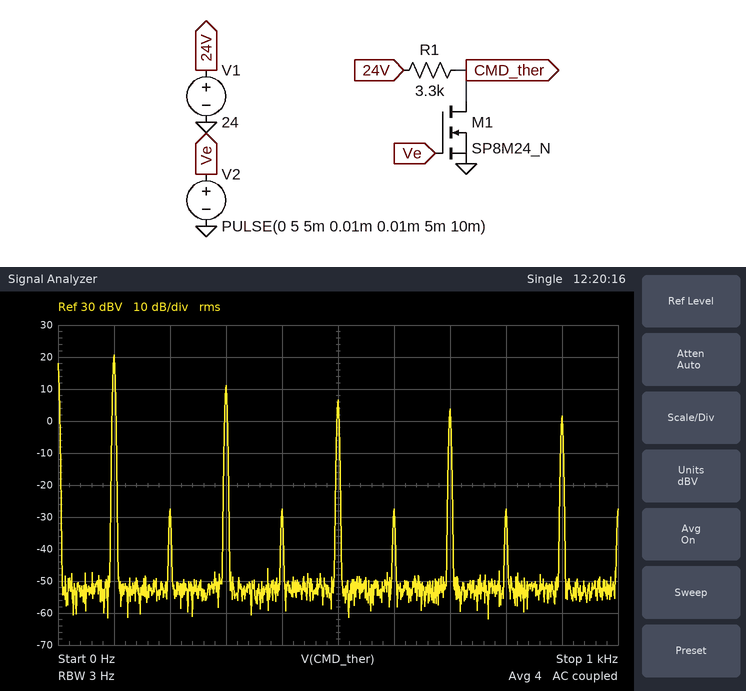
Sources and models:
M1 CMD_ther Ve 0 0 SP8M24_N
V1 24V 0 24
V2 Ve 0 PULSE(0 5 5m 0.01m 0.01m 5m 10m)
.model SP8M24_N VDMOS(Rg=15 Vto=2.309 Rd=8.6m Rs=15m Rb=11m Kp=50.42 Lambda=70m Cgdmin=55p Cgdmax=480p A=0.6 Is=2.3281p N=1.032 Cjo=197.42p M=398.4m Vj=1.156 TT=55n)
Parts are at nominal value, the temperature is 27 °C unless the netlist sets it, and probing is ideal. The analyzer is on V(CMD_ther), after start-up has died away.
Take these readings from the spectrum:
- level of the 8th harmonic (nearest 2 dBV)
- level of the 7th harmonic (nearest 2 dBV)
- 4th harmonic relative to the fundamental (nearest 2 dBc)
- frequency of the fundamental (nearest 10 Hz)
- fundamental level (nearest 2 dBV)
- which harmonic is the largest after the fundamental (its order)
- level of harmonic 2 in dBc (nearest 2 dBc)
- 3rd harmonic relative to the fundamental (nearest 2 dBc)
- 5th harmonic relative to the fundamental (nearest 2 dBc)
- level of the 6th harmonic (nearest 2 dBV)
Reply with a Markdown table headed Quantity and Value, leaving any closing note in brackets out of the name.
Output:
| Quantity | Value |
|---|---|
| level of the 8th harmonic | -28 dBV |
| level of the 7th harmonic | 4 dBV |
| 4th harmonic relative to the fundamental | -48 dBc |
| frequency of the fundamental | 100 Hz |
| fundamental level | 20 dBV |
| which harmonic is the largest after the fundamental | 3 |
| level of harmonic 2 in dBc | -48 dBc |
| 3rd harmonic relative to the fundamental | -10 dBc |
| 5th harmonic relative to the fundamental | -14 dBc |
| level of the 6th harmonic | -28 dBV |
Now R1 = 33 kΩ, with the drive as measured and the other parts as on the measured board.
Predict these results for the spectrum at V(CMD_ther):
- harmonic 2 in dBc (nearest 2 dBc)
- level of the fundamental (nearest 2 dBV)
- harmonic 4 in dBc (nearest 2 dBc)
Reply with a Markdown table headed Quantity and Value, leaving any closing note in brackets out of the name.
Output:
| Quantity | Value |
|---|---|
| harmonic 2 in dBc | -44 dBc |
| level of the fundamental | 20 dBV |
| harmonic 4 in dBc | -44 dBc |
